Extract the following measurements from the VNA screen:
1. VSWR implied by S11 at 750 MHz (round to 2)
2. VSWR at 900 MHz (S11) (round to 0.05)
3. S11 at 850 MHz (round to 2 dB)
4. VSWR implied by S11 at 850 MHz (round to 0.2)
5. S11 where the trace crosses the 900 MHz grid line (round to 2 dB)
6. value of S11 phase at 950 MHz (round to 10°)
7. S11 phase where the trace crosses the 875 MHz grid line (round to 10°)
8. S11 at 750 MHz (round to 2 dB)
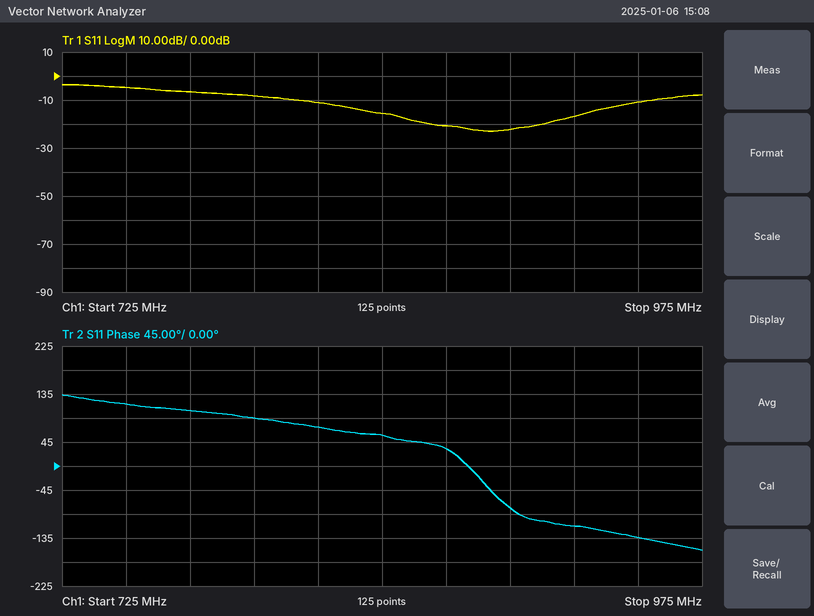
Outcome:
4
1.15
-16 dB
1.4
-22 dB
-130°
30°
-4 dB
